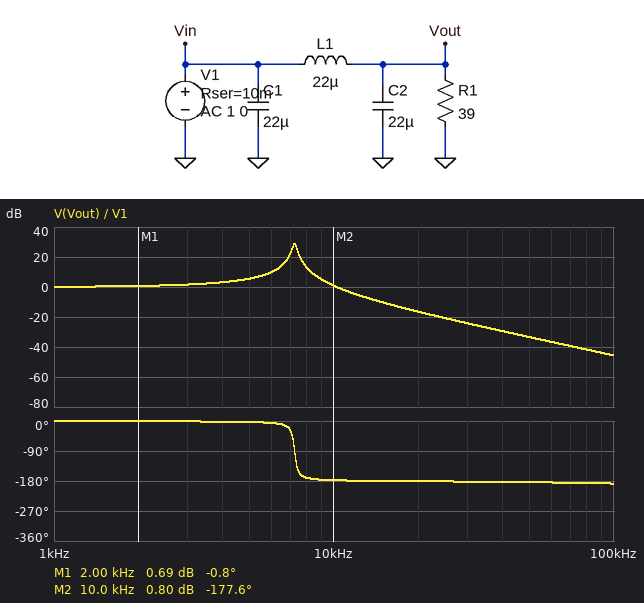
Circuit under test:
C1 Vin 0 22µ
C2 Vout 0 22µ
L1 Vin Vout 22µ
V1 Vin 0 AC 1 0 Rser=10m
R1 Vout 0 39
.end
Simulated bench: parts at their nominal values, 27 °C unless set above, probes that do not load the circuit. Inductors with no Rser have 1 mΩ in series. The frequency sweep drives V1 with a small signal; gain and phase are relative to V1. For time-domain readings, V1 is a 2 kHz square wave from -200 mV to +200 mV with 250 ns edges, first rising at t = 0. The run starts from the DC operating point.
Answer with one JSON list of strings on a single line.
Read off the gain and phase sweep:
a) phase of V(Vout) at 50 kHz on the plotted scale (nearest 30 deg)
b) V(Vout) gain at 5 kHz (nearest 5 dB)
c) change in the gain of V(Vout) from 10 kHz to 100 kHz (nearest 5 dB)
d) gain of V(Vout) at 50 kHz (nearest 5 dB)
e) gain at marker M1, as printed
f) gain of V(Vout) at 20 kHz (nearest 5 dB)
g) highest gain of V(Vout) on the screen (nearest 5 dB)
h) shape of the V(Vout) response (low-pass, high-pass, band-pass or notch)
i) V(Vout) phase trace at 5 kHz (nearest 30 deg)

["-180 deg", "5 dB", "-45 dB", "-35 dB", "0.69 dB", "-15 dB", "30 dB", "low-pass", "0 deg"]
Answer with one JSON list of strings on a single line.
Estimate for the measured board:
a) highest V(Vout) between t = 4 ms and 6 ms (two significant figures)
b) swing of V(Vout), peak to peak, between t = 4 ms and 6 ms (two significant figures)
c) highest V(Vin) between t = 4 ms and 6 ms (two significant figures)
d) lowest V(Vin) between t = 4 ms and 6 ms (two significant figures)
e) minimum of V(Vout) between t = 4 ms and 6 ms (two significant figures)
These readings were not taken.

["460 mV", "920 mV", "200 mV", "-200 mV", "-460 mV"]
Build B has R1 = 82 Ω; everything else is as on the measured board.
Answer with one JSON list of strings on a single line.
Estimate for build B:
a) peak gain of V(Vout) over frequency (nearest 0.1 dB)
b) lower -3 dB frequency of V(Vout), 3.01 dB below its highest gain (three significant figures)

["32.7 dB", "7.15 kHz"]
